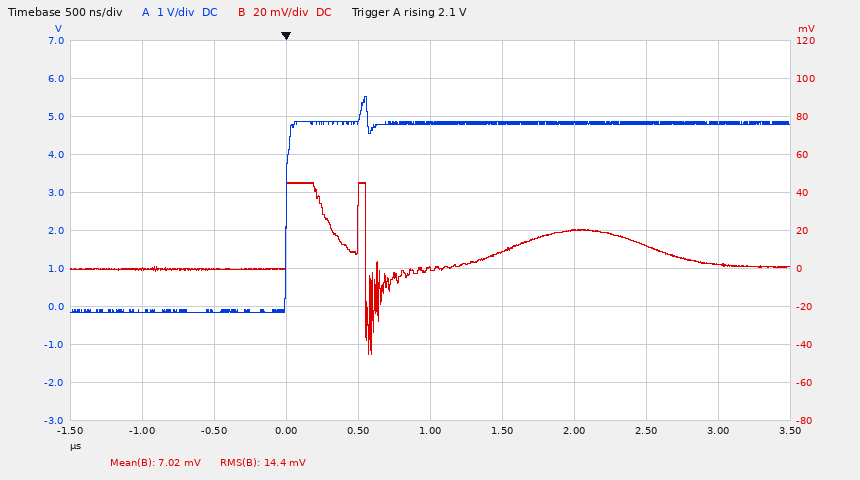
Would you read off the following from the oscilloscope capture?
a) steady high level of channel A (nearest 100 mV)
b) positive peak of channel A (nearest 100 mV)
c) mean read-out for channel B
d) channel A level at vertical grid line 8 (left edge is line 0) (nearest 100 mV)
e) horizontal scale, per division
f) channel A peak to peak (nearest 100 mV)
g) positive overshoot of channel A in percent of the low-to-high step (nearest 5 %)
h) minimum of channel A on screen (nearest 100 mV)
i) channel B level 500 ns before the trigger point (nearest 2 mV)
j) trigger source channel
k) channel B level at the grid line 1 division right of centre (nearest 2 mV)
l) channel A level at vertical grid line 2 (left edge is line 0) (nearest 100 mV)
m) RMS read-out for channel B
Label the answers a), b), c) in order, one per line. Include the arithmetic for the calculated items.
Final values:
a) 4.8 V
b) 5.5 V
c) 7.02 mV
d) 4.8 V
e) 500 ns
f) 5.5 V − (-200 mV) = 5.7 V
g) 15 %
h) -200 mV
i) 0 mV
j) channel A
k) 8 mV
l) -100 mV
m) 14.4 mV
